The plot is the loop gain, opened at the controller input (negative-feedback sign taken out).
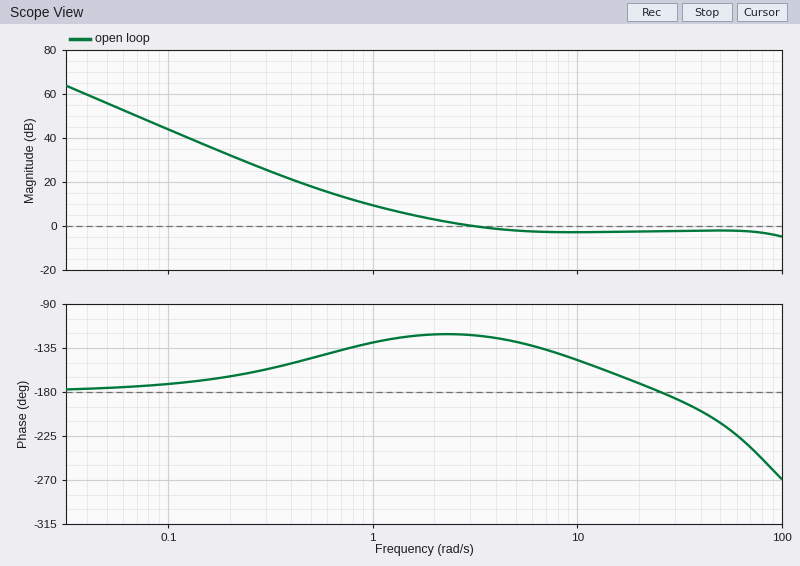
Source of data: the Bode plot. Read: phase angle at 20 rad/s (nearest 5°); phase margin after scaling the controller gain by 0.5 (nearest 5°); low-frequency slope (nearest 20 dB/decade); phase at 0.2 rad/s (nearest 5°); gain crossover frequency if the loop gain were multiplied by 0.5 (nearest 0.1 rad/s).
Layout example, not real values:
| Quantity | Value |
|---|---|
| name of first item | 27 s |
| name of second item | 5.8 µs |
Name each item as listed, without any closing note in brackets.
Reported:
| Quantity | Value |
|---|---|
| phase angle at 20 rad/s | -170° |
| phase margin after scaling the controller gain by 0.5 | 55° |
| low-frequency slope | -40 dB/decade |
| phase at 0.2 rad/s | -165° |
| gain crossover frequency if the loop gain were multiplied by 0.5 | 1.4 rad/s |
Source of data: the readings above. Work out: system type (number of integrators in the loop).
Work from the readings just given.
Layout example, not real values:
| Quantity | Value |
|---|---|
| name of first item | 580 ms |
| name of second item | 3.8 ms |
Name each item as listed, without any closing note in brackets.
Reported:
| Quantity | Value |
|---|---|
| system type | 2 |
